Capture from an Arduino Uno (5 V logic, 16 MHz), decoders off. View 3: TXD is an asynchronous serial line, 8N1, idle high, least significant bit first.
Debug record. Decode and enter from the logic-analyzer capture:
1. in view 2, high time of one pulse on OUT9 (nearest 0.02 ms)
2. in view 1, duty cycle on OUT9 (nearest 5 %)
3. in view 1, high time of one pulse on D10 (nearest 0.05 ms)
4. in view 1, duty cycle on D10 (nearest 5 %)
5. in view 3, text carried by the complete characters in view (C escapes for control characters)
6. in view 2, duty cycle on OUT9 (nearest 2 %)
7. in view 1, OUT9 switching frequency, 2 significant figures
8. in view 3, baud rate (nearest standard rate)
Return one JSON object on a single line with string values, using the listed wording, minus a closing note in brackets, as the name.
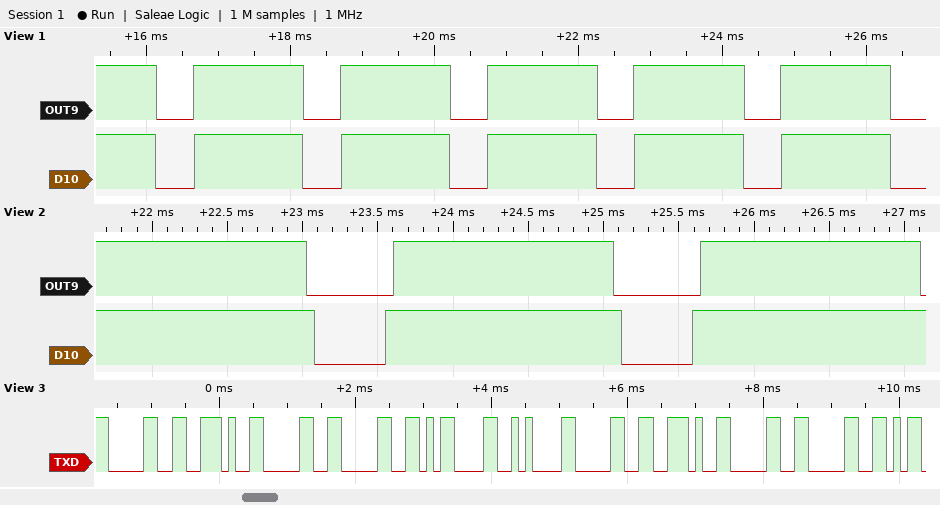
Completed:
{"in view 2, high time of one pulse on OUT9": "1.46 ms", "in view 1, duty cycle on OUT9": "75 %", "in view 1, high time of one pulse on D10": "1.50 ms", "in view 1, duty cycle on D10": "75 %", "in view 3, text carried by the complete characters in view": "\"0.00\\r\\n0.00\"", "in view 2, duty cycle on OUT9": "72 %", "in view 1, OUT9 switching frequency, 2 significant figures": "490 Hz", "in view 3, baud rate": "9600 baud"}
